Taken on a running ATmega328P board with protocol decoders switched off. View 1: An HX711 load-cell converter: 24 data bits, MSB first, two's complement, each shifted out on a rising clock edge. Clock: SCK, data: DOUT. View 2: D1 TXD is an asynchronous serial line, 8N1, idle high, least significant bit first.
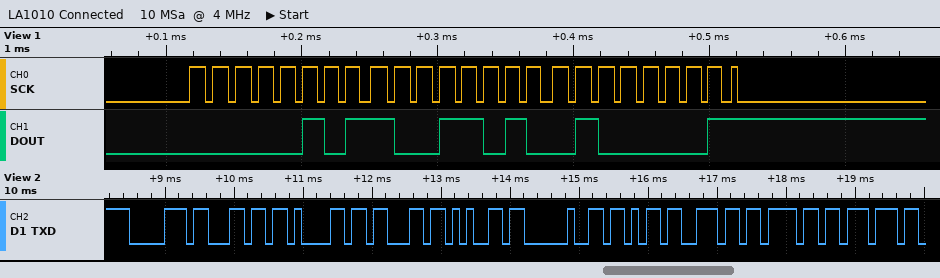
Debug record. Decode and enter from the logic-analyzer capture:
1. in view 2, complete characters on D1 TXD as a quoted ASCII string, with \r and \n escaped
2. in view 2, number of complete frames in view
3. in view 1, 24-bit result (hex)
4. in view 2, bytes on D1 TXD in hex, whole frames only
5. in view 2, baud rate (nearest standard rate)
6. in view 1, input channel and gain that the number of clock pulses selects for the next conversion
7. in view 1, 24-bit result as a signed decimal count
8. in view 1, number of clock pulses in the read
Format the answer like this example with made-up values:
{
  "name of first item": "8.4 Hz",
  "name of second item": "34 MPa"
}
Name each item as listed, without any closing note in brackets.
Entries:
{
  "in view 2, complete characters on D1 TXD as a quoted ASCII string, with \\r and \\n escaped": "\"place know\"",
  "in view 2, number of complete frames in view": "10",
  "in view 1, 24-bit result": "0x059A41",
  "in view 2, bytes on D1 TXD in hex, whole frames only": "70 6C 61 63 65 20 6B 6E 6F 77",
  "in view 2, baud rate": "9600 baud",
  "in view 1, input channel and gain that the number of clock pulses selects for the next conversion": "channel A, gain 128",
  "in view 1, 24-bit result as a signed decimal count": "367169",
  "in view 1, number of clock pulses in the read": "25"
}
